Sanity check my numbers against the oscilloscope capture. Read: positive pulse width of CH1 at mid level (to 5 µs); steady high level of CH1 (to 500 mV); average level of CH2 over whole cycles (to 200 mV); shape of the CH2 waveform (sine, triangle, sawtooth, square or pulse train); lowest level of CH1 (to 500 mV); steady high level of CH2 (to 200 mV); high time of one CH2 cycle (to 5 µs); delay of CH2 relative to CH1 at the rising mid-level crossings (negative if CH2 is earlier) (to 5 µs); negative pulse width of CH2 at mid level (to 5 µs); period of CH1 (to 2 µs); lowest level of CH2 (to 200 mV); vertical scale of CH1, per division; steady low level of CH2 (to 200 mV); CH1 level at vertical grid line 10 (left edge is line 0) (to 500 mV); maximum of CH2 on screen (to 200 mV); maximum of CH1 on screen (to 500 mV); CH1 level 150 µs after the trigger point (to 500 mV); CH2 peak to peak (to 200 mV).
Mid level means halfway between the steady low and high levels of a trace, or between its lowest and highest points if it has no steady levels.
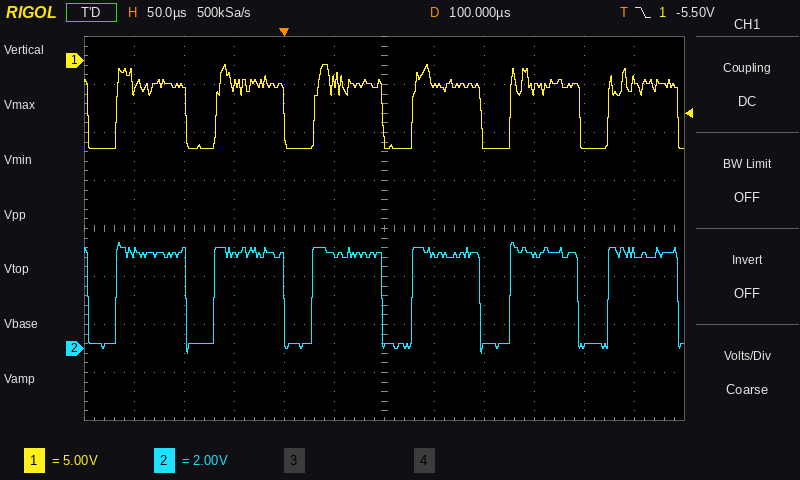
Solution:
70 µs
-2.5 V
2.8 V
pulse train
-9.0 V
4.0 V
70 µs
0 µs
30 µs
98 µs
-200 mV
5 V
200 mV
-9.0 V
4.4 V
-500 mV
-2.5 V
4.6 V
